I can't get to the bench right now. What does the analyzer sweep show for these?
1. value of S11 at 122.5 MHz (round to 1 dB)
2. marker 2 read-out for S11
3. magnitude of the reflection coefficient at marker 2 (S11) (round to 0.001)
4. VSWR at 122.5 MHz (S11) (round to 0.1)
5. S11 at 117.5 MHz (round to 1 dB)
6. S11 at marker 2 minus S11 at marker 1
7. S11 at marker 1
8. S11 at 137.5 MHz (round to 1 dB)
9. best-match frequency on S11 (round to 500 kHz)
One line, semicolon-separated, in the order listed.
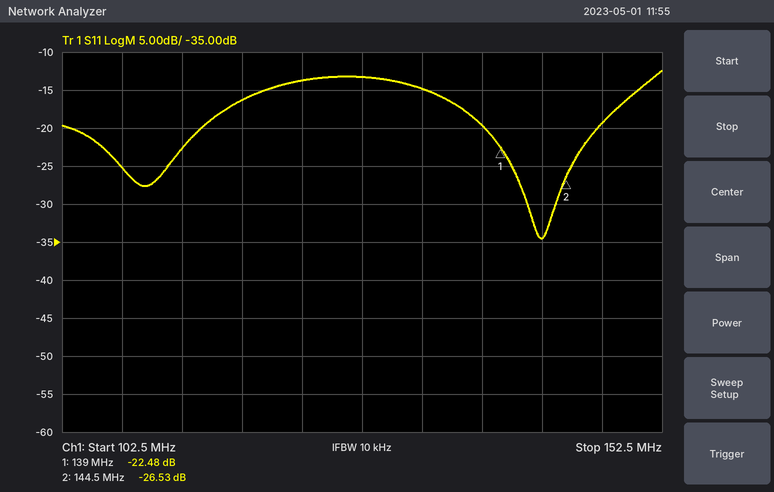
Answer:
-14 dB; -26.53 dB; 0.047; 1.5; -16 dB; -4.05 dB; -22.48 dB; -20 dB; 142.5 MHz
